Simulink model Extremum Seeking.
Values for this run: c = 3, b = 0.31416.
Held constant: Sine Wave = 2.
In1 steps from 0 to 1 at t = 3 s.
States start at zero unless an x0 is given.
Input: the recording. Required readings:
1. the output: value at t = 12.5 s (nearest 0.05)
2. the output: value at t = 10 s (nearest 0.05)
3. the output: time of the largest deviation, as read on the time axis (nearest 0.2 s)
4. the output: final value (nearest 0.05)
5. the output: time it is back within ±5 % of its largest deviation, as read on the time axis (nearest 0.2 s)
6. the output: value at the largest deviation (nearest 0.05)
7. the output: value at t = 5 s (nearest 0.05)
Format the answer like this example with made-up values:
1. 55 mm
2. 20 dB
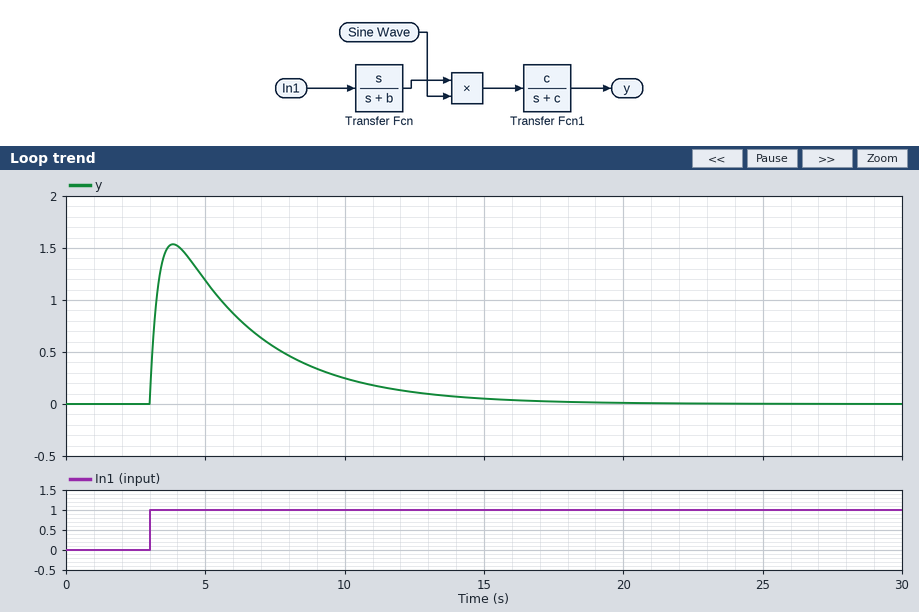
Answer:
1. 0.10
2. 0.25
3. 3.8 s
4. 0.00
5. 13.8 s
6. 1.55
7. 1.20
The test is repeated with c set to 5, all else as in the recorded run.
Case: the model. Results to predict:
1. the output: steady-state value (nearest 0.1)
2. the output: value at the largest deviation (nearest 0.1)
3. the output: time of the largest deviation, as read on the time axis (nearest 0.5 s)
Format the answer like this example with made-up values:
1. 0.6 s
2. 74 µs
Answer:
1. 0.0
2. 1.7
3. 3.5 s
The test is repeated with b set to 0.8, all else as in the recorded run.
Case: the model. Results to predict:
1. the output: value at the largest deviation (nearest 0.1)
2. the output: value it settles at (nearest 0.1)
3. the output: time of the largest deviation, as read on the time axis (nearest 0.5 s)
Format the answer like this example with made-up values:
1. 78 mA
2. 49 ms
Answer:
1. 1.2
2. 0.0
3. 3.5 s
